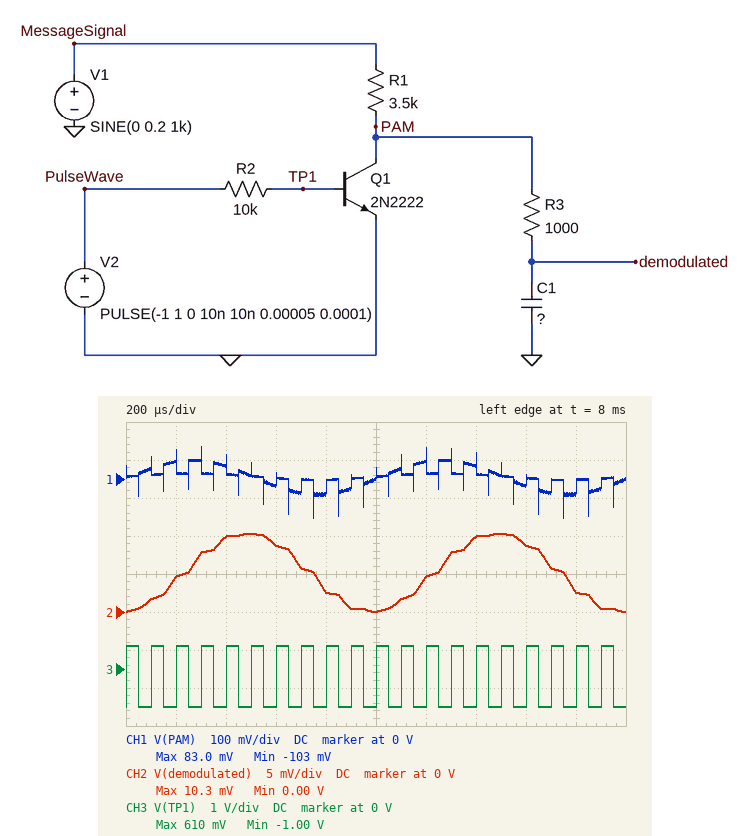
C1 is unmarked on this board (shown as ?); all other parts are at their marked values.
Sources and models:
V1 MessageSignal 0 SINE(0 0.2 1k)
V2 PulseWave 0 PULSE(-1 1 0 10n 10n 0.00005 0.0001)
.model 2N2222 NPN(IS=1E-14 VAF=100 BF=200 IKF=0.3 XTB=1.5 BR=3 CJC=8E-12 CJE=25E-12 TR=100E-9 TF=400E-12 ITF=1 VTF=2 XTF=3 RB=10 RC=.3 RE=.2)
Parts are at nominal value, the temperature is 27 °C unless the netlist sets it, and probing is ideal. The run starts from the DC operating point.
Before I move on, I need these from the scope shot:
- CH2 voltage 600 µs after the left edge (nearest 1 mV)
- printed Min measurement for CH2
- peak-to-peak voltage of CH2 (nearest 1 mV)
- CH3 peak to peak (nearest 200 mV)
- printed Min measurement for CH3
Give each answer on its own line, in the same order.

9 mV
0.00 V
10 mV
1.6 V
-1.00 V
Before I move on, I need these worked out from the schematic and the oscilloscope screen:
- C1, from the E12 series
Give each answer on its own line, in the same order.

820 nF
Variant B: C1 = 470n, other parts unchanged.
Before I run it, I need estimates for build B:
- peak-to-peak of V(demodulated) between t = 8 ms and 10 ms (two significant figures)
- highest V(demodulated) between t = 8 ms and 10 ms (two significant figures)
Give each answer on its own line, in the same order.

18 mV
14 mV
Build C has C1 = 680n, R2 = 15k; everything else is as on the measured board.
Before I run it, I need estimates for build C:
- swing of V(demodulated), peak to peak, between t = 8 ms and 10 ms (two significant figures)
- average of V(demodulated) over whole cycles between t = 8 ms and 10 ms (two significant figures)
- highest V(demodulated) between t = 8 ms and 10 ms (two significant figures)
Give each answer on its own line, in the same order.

13 mV
4.7 mV
11 mV
